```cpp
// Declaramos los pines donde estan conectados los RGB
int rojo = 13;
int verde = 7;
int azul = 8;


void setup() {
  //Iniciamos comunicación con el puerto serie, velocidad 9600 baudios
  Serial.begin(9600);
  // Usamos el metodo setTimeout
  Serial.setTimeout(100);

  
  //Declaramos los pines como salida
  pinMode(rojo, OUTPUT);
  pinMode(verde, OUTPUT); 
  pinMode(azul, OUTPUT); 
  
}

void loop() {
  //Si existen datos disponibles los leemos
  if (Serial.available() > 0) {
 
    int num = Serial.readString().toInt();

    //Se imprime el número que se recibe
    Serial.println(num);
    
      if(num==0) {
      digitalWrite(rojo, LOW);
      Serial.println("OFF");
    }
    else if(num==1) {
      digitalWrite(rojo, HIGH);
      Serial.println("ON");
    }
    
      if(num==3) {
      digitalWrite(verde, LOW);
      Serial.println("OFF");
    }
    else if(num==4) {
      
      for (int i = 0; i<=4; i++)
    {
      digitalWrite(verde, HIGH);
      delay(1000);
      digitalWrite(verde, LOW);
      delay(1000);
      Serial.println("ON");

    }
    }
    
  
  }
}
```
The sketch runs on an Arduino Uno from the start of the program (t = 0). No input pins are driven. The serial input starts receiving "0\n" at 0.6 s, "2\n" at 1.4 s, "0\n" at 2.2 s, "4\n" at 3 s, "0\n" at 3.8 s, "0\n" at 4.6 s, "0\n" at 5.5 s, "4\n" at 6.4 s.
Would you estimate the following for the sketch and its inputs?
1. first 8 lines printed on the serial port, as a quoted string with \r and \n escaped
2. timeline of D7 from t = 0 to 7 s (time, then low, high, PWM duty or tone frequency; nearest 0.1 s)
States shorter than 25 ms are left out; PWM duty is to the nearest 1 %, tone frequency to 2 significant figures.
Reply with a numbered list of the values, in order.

1. "0\r\nOFF\r\n2\r\n0\r\nOFF\r\n4\r\nON\r\nON\r\n"
2. 0 s low; 3.1 s high; 4.1 s low; 5.1 s high; 6.1 s low
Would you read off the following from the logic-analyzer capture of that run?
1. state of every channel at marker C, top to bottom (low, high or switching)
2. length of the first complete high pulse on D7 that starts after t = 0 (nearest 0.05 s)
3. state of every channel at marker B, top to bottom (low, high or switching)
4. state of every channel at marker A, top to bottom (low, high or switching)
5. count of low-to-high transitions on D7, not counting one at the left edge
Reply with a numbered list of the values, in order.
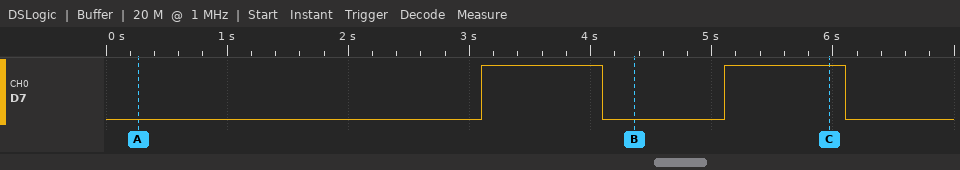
1. D7 high
2. 1.00 s
3. D7 low
4. D7 low
5. 2
